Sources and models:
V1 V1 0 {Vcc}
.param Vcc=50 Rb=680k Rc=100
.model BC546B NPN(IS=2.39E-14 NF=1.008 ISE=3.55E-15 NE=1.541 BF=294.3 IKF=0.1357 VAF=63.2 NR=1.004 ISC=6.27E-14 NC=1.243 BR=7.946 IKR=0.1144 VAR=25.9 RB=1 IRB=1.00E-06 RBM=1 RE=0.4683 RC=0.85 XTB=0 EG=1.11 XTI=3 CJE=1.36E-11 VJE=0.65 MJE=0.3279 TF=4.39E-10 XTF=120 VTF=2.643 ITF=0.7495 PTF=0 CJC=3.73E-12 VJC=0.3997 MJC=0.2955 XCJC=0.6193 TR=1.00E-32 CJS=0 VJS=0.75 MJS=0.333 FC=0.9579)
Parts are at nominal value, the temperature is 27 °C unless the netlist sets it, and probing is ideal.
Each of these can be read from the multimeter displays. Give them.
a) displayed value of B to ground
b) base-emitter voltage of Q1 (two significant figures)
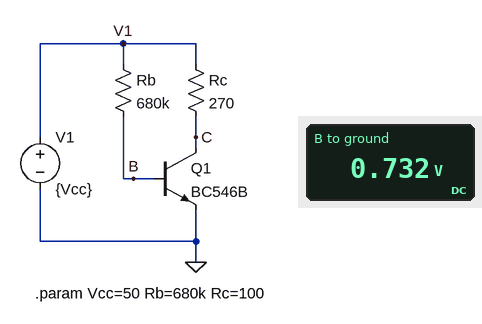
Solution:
0.732 V
730 mV
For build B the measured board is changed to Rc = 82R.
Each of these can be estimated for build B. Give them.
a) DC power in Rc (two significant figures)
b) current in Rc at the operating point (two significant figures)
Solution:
84 mW
32 mA
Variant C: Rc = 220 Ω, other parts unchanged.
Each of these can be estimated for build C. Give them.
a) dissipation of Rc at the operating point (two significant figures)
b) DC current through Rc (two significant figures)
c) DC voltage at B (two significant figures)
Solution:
210 mW
31 mA
730 mV
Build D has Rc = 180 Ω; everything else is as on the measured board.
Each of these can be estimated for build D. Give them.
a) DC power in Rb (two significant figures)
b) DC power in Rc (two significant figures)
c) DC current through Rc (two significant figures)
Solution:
3.6 mW
170 mW
31 mA
